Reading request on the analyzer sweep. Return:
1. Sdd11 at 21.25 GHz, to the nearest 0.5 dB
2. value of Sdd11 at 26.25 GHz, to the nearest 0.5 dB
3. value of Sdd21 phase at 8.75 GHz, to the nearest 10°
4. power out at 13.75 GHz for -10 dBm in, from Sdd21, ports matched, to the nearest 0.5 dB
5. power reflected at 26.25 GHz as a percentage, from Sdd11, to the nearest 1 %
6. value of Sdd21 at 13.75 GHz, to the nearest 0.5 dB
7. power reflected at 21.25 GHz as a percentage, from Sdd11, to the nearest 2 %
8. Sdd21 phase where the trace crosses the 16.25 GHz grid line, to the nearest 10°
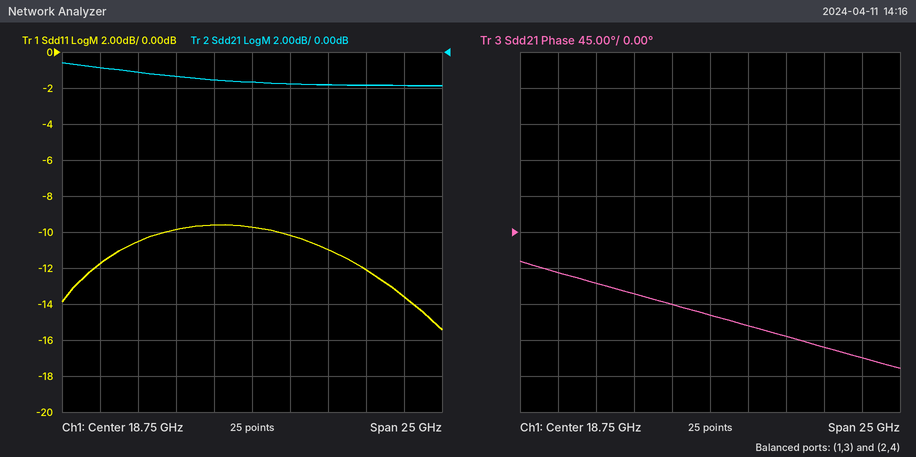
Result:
-10.0 dB
-12.0 dB
-50°
-11.5 dBm
6 %
-1.5 dB
10 %
-90°
